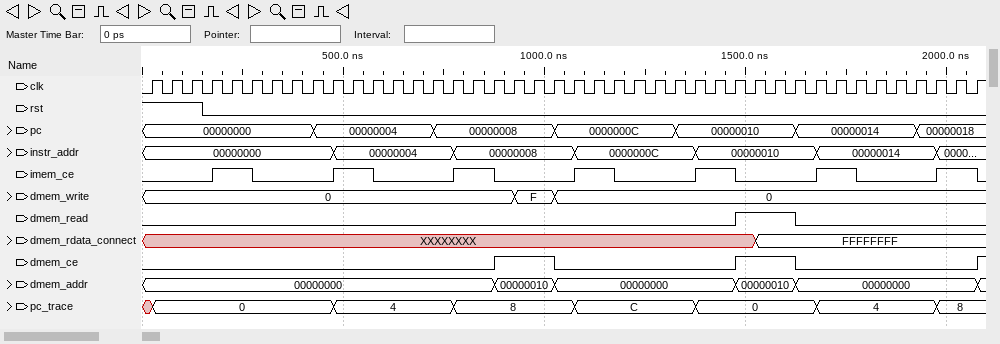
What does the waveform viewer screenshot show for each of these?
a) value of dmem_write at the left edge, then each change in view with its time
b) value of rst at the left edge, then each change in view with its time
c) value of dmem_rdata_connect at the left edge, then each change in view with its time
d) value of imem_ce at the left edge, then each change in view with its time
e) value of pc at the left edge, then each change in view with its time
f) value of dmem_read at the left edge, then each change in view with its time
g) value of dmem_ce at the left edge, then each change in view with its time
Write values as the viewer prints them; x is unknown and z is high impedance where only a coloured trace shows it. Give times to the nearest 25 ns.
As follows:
0, F at 925 ns, 0 at 1025 ns
1, 0 at 150 ns
XXXXXXXX, FFFFFFFF at 1525 ns
0, 1 at 175 ns, 0 at 275 ns, 1 at 475 ns, 0 at 575 ns, 1 at 775 ns, 0 at 875 ns, 1 at 1075 ns, 0 at 1175 ns, 1 at 1375 ns, 0 at 1475 ns, 1 at 1675 ns, 0 at 1775 ns, 1 at 1975 ns, 0 at 2075 ns
00000000, 00000004 at 425 ns, 00000008 at 725 ns, 0000000C at 1025 ns, 00000010 at 1325 ns, 00000014 at 1625 ns, 00000018 at 1925 ns
0, 1 at 1475 ns, 0 at 1625 ns
0, 1 at 875 ns, 0 at 1025 ns, 1 at 1475 ns, 0 at 1625 ns, 1 at 2075 ns
